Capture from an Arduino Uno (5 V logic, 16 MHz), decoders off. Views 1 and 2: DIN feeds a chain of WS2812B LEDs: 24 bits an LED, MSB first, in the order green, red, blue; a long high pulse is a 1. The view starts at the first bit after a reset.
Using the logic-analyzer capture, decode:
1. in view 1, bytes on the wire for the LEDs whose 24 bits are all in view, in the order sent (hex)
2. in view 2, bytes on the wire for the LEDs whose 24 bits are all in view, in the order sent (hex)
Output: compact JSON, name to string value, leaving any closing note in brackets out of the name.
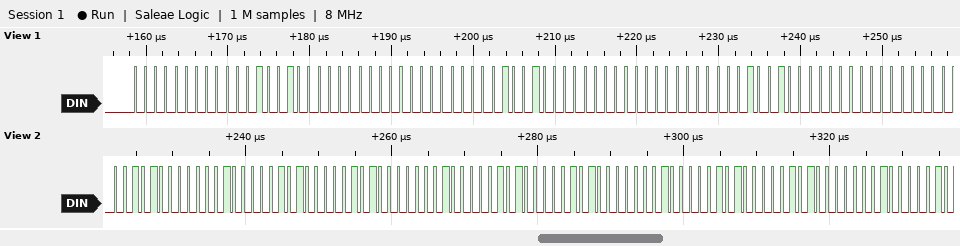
{"in view 1, bytes on the wire for the LEDs whose 24 bits are all in view, in the order sent": "00 09 00 00 09 00 00 09 00", "in view 2, bytes on the wire for the LEDs whose 24 bits are all in view, in the order sent": "28 08 28 28 08 28 28 08 28"}
